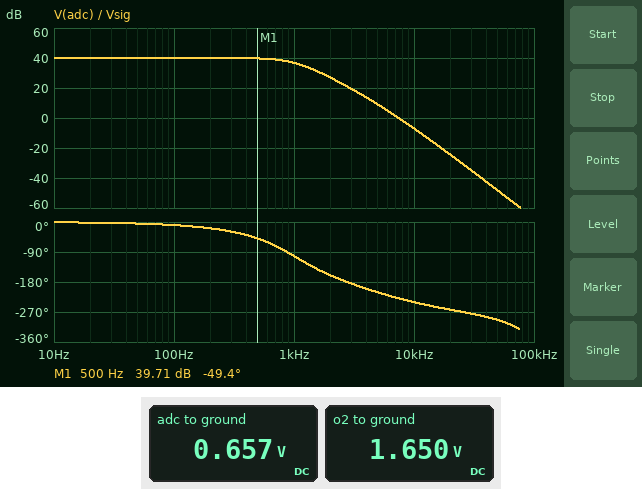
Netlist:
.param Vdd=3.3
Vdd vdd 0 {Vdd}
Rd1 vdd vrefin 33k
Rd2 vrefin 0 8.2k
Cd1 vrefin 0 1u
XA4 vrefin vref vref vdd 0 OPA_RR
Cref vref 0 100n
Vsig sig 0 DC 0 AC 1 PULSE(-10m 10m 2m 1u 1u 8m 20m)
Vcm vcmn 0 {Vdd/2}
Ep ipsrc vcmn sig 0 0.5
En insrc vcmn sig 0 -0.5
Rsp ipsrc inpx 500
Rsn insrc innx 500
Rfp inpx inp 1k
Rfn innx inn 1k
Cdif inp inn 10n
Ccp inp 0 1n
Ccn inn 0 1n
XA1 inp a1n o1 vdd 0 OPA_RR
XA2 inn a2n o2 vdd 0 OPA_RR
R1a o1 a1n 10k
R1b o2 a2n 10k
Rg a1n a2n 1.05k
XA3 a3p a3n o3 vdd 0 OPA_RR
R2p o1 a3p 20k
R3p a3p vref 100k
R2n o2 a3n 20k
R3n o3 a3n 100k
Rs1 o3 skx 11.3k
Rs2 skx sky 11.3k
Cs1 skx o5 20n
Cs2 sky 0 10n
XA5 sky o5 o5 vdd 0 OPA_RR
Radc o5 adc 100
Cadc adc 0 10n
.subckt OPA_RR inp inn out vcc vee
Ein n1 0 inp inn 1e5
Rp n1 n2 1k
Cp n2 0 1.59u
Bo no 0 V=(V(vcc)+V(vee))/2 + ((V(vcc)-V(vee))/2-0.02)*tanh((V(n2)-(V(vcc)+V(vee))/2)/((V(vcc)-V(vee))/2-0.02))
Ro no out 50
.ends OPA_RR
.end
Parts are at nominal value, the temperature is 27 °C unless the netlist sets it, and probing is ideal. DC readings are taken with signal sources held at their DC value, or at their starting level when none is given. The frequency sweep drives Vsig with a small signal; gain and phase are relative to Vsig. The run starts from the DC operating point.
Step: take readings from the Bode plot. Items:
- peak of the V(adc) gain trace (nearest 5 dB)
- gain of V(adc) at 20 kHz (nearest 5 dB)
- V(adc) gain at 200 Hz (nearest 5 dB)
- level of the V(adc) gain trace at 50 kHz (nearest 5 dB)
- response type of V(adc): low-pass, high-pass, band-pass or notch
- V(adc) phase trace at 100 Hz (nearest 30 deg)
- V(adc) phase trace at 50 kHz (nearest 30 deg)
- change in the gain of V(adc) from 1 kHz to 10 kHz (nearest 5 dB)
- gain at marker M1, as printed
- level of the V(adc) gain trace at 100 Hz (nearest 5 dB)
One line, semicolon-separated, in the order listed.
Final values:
40 dB; -25 dB; 40 dB; -50 dB; low-pass; 0 deg; -300 deg; -45 dB; 39.71 dB; 40 dB
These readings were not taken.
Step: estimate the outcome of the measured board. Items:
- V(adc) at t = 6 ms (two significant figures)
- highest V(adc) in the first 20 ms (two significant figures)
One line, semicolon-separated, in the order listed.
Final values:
1.7 V; 1.7 V
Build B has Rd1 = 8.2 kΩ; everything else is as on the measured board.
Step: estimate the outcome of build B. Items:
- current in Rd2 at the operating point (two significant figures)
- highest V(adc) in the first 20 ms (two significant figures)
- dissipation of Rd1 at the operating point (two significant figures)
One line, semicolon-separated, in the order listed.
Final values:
200 µA; 2.7 V; 330 µW
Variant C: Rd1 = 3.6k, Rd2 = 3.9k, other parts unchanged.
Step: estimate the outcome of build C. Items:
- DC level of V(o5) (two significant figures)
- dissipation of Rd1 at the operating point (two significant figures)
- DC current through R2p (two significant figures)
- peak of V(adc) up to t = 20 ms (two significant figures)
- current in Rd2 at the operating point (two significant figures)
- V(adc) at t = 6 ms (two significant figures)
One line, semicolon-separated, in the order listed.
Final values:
1.7 V; 700 µW; 550 nA; 2.8 V; 440 µA; 2.7 V
